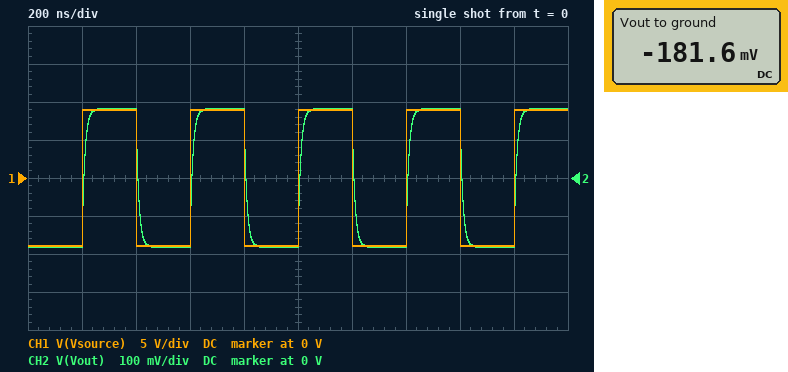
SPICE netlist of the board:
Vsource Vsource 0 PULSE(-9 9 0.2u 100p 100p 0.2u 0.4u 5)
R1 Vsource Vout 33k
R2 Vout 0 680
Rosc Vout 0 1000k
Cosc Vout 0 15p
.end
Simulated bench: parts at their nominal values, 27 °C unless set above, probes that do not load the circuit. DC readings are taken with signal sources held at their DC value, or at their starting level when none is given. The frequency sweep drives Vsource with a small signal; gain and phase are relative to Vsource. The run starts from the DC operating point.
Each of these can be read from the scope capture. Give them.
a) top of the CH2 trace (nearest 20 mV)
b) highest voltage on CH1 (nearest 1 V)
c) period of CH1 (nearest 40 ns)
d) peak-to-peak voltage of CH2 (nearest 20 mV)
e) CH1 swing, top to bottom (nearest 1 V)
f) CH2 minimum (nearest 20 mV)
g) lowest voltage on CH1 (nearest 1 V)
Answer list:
180 mV
9 V
400 ns
360 mV
18 V
-180 mV
-9 V
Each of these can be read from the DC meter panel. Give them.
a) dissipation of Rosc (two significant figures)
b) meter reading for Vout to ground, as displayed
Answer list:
33 nW
-181.6 mV
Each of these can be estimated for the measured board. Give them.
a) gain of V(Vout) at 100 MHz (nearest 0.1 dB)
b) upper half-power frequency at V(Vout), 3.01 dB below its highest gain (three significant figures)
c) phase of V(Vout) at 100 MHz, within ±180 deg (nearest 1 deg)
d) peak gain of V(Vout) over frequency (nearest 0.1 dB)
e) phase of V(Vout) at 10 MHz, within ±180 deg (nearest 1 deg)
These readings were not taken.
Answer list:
-50.0 dB
15.9 MHz
-81 deg
-33.9 dB
-32 deg
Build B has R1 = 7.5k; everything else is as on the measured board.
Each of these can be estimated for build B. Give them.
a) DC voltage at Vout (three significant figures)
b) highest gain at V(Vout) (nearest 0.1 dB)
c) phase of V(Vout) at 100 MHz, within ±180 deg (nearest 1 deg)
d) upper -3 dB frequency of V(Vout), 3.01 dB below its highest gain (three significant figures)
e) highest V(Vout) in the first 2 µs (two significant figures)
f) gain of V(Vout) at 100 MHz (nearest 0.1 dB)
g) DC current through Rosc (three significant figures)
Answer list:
-748 mV
-21.6 dB
-80 deg
17.0 MHz
750 mV
-37.1 dB
748 nA
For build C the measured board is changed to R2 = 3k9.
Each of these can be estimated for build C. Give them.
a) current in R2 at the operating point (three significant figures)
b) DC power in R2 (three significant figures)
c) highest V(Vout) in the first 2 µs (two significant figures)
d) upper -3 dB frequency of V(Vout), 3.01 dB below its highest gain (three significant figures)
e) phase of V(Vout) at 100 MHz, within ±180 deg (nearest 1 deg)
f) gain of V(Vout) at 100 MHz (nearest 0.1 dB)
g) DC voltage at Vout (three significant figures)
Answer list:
243 µA
230 µW
910 mV
3.05 MHz
-88 deg
-49.9 dB
-948 mV
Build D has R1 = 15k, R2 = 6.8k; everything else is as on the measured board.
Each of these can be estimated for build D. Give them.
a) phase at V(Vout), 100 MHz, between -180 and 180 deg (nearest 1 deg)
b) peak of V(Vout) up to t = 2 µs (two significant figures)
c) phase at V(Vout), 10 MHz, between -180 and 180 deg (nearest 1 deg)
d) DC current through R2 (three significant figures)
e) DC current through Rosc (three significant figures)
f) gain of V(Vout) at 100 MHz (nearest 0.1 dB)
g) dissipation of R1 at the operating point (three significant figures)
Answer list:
-89 deg
2.5 V
-77 deg
411 µA
2.79 µA
-43.0 dB
2.57 mW
